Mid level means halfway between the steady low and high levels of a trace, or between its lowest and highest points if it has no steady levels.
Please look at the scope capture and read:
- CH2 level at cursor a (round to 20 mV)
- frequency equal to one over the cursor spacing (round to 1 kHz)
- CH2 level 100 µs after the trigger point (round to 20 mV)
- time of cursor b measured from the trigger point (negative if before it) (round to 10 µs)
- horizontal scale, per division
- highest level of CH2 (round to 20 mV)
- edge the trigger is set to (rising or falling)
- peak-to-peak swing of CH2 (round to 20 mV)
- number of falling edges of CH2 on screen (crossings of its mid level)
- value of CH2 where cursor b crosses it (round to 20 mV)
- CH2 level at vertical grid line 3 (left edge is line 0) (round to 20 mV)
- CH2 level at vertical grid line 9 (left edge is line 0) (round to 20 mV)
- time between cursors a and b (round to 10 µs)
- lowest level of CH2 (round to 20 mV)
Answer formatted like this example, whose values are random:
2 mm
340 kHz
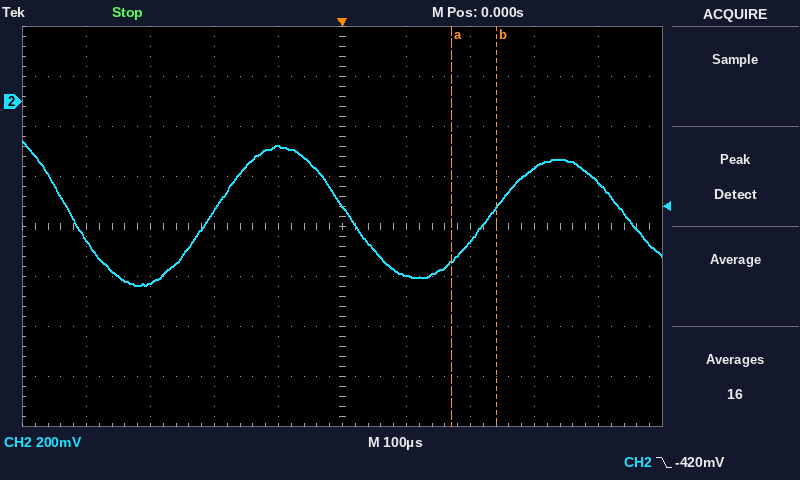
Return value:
-640 mV
14 kHz
-700 mV
+240 µs
100 µs
-160 mV
falling
580 mV
3
-420 mV
-440 mV
-320 mV
70 µs
-740 mV
